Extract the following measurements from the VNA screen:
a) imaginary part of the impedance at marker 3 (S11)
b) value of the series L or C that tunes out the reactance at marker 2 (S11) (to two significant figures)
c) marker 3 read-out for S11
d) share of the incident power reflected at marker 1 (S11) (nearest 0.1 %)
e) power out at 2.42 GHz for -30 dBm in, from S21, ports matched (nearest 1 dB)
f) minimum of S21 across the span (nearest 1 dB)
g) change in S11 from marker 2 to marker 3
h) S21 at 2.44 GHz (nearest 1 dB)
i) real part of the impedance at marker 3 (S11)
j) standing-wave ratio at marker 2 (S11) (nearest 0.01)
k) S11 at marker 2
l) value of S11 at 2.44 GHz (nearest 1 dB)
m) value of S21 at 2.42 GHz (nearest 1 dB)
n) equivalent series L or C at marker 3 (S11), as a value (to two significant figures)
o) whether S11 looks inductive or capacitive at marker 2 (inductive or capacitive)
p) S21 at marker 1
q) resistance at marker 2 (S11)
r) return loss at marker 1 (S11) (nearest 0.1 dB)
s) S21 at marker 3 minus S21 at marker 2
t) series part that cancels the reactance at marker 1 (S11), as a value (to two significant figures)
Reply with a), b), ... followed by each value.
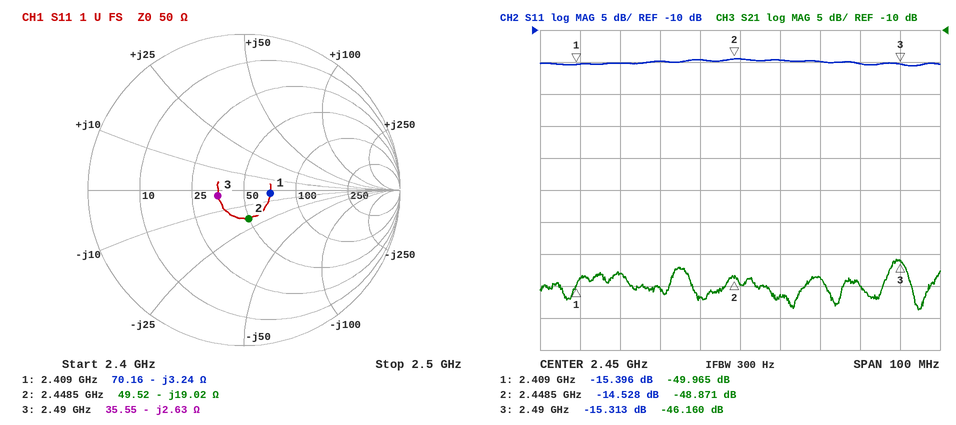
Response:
a) -2.63 Ω
b) 1.2 nH
c) -15.313 dB
d) 2.9 %
e) -78 dBm
f) -54 dB
g) -0.785 dB
h) -52 dB
i) 35.55 Ω
j) 1.46
k) -14.528 dB
l) -15 dB
m) -48 dB
n) 24 pF
o) capacitive
p) -49.965 dB
q) 49.52 Ω
r) 15.4 dB
s) 2.711 dB
t) 210 pH
